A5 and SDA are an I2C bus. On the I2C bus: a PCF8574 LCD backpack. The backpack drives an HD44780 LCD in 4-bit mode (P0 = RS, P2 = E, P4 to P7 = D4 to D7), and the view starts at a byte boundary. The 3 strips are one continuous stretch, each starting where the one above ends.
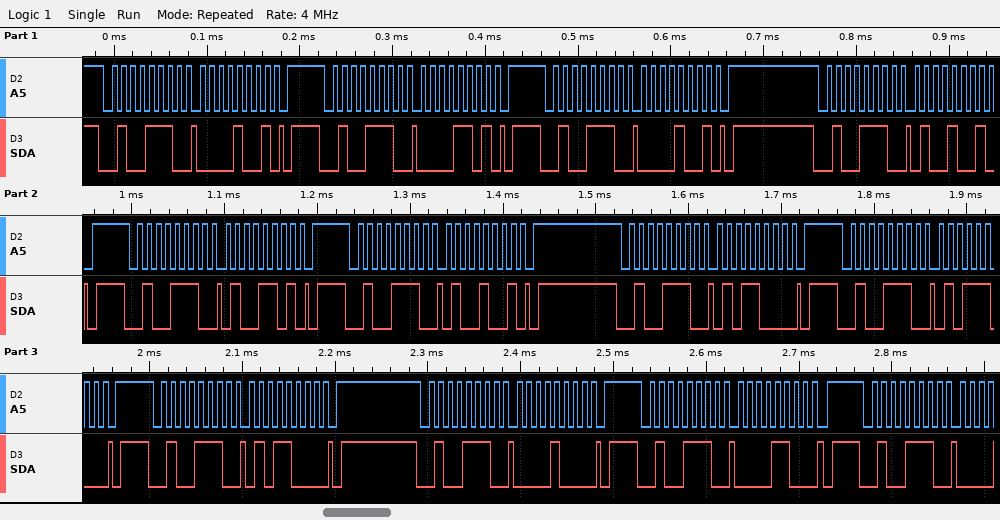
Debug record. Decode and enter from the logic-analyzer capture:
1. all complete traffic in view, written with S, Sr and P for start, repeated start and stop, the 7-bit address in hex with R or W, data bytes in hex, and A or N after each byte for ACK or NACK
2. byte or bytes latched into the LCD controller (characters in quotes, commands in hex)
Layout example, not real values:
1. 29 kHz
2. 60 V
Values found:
1. S 27W A 09 A P S 27W A 0D A P S 27W A 09 A P S 27W A 49 A P S 27W A 4D A P S 27W A 49 A P S 27W A 58 A P S 27W A 5C A P S 27W A 58 A P S 27W A 08 A P S 27W A 0C A P S 27W A
2. data 0x04
